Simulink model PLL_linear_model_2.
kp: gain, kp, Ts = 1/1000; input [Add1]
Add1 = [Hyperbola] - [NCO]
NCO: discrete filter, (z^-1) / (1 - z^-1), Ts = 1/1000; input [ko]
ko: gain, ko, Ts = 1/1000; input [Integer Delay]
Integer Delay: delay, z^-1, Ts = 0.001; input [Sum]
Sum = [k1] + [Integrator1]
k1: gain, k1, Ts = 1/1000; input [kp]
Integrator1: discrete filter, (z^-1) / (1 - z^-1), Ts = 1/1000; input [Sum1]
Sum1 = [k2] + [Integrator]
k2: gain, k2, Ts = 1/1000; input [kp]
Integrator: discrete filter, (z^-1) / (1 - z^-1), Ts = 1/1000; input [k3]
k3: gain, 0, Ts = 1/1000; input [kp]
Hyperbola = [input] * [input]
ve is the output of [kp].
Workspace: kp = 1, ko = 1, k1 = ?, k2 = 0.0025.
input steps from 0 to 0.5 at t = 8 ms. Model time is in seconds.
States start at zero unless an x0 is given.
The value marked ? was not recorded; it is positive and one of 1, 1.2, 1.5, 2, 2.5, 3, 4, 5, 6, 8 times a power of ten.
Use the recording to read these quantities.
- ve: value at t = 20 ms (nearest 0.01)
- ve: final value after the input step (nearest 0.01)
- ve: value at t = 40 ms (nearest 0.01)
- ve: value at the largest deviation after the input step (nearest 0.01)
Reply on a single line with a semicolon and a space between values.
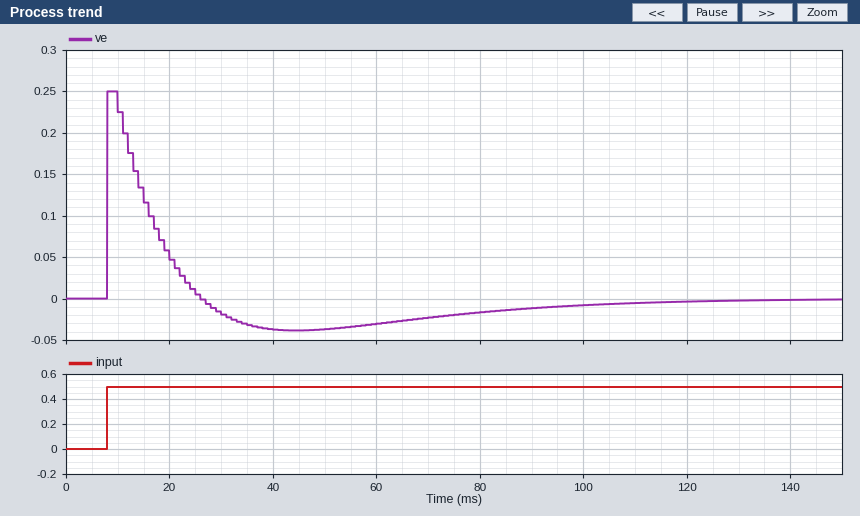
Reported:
0.05; 0.00; -0.04; 0.25
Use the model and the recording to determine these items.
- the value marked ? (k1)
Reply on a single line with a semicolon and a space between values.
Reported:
0.1
